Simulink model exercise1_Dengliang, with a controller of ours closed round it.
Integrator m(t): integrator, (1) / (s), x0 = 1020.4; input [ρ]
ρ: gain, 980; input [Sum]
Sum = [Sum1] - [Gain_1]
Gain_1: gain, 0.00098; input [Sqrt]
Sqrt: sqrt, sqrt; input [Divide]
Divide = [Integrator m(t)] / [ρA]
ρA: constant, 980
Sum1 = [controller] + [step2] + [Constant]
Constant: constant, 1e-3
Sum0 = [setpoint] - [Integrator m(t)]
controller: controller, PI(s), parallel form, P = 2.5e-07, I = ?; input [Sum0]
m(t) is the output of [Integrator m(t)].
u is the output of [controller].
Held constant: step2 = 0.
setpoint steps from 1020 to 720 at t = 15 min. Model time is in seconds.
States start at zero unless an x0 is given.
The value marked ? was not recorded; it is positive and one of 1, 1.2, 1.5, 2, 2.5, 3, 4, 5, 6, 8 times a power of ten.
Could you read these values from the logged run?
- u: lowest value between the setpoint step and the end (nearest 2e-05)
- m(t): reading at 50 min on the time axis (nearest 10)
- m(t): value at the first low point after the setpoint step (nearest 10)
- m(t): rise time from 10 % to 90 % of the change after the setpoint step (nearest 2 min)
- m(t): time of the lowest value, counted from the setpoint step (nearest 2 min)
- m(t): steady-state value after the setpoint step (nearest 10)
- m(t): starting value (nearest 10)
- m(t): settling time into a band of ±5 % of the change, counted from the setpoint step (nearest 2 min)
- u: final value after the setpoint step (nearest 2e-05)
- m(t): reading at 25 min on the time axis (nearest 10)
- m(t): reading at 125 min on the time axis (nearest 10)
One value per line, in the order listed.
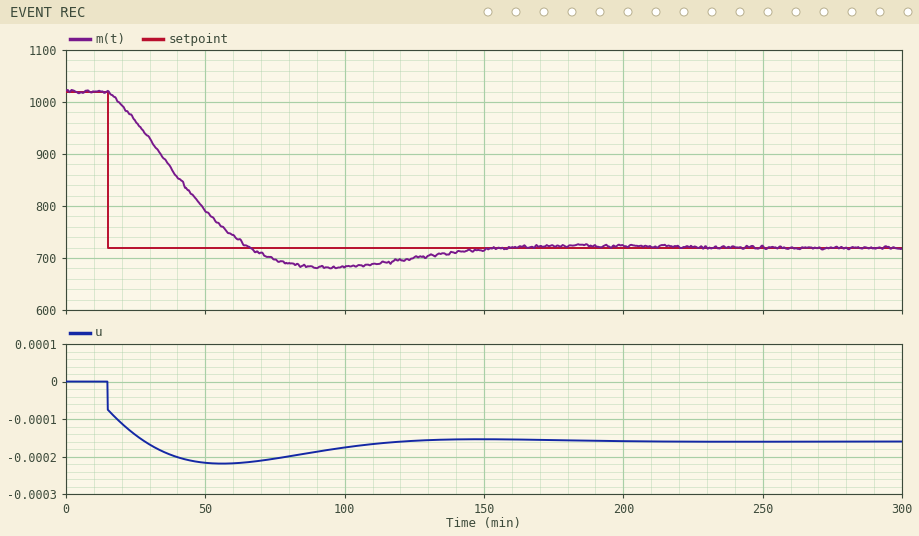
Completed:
-0.00022
790
680
38 min
78 min
720
1020
116 min
-0.00016
960
700
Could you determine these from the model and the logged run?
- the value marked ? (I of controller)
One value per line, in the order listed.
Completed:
5e-10
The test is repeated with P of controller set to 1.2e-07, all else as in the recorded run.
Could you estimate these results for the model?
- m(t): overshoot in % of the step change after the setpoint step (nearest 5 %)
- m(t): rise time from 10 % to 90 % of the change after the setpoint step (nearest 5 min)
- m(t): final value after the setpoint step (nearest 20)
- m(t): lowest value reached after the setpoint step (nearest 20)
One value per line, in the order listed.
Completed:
20 %
35 min
720
660
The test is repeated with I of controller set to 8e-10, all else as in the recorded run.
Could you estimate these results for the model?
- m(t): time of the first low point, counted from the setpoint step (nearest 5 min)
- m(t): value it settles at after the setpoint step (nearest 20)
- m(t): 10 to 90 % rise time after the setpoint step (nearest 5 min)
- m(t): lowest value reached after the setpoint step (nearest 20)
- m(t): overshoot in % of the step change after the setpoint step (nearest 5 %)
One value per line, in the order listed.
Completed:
60 min
720
25 min
660
20 %
